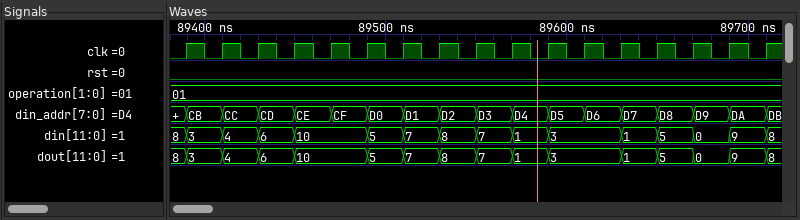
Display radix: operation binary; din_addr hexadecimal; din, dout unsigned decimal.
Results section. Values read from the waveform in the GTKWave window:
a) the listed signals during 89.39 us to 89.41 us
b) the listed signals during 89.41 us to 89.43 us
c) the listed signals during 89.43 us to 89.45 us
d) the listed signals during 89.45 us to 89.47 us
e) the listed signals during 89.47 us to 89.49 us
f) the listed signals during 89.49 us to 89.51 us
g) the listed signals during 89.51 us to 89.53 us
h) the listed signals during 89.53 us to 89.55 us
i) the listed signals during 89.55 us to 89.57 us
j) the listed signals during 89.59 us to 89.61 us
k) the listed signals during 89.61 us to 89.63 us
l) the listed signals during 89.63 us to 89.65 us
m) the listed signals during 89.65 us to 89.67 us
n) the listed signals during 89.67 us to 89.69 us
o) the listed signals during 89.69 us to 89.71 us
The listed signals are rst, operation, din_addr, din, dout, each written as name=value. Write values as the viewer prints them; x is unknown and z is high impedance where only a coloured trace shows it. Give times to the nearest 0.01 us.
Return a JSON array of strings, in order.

["rst=0, operation=01, din_addr=CB, din=3, dout=3", "rst=0, operation=01, din_addr=CC, din=4, dout=4", "rst=0, operation=01, din_addr=CD, din=6, dout=6", "rst=0, operation=01, din_addr=CE, din=10, dout=10", "rst=0, operation=01, din_addr=CF, din=10, dout=10", "rst=0, operation=01, din_addr=D0, din=5, dout=5", "rst=0, operation=01, din_addr=D1, din=7, dout=7", "rst=0, operation=01, din_addr=D2, din=8, dout=8", "rst=0, operation=01, din_addr=D3, din=7, dout=7", "rst=0, operation=01, din_addr=D5, din=3, dout=3", "rst=0, operation=01, din_addr=D6, din=3, dout=3", "rst=0, operation=01, din_addr=D7, din=1, dout=1", "rst=0, operation=01, din_addr=D8, din=5, dout=5", "rst=0, operation=01, din_addr=D9, din=0, dout=0", "rst=0, operation=01, din_addr=DA, din=9, dout=9"]
